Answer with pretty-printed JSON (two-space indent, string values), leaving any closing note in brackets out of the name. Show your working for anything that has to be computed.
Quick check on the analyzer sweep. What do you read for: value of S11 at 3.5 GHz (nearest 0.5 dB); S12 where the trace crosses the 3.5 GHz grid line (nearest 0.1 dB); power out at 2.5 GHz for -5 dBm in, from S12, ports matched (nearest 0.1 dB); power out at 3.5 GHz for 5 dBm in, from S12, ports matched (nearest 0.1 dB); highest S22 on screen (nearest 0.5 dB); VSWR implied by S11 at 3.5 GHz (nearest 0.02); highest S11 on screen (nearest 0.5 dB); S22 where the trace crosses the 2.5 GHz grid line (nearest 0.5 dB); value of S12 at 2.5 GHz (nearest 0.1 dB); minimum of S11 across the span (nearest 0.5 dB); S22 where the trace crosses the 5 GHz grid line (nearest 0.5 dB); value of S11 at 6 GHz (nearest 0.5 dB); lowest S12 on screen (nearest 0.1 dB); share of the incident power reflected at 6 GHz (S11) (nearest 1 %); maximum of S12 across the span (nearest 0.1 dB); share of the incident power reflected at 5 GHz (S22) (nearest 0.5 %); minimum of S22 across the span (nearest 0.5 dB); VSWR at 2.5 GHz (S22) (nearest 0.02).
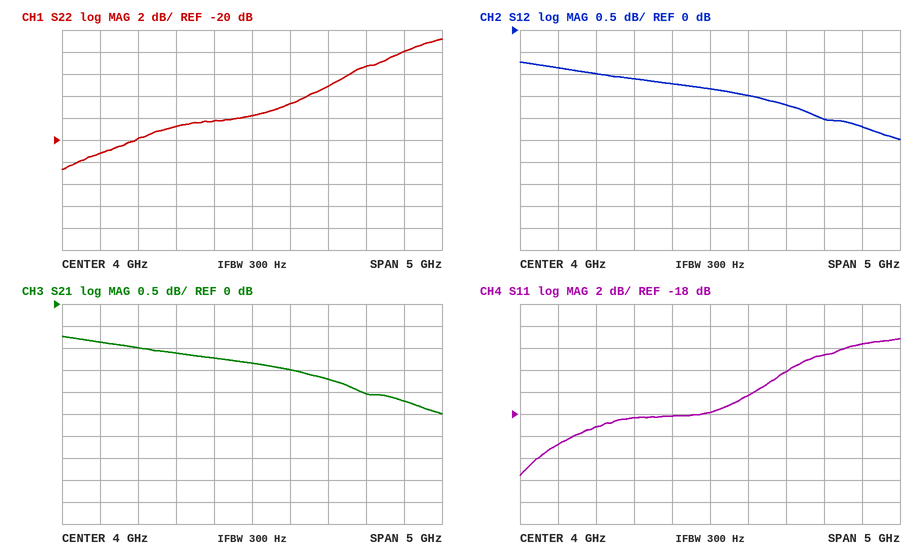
{
  "value of S11 at 3.5 GHz": "-18.0 dB",
  "S12 where the trace crosses the 3.5 GHz grid line": "-1.2 dB",
  "power out at 2.5 GHz for -5 dBm in, from S12, ports matched": "-5 dBm + (-1.0 dB) = -6.0 dBm",
  "power out at 3.5 GHz for 5 dBm in, from S12, ports matched": "5 dBm + (-1.2 dB) = 3.8 dBm",
  "highest S22 on screen": "-11.0 dB",
  "VSWR implied by S11 at 3.5 GHz": "|Γ| = 10^(-18/20) = 0.1259; VSWR = (1 + 0.1259)/(1 − 0.1259) ≈ 1.29, so 1.28 to the nearest 0.02",
  "highest S11 on screen": "-11.0 dB",
  "S22 where the trace crosses the 2.5 GHz grid line": "-20.0 dB",
  "value of S12 at 2.5 GHz": "-1.0 dB",
  "minimum of S11 across the span": "-23.5 dB",
  "S22 where the trace crosses the 5 GHz grid line": "-15.0 dB",
  "value of S11 at 6 GHz": "-11.5 dB",
  "lowest S12 on screen": "-2.5 dB",
  "share of the incident power reflected at 6 GHz (S11)": "10^(-11.5/10) ≈ 7 %",
  "maximum of S12 across the span": "-0.7 dB",
  "share of the incident power reflected at 5 GHz (S22)": "10^(-15/10) ≈ 3.16 %, so 3.0 % to the nearest 0.5 %",
  "minimum of S22 across the span": "-22.5 dB",
  "VSWR at 2.5 GHz (S22)": "|Γ| = 10^(-20/20) = 0.1000; VSWR = (1 + 0.1000)/(1 − 0.1000) ≈ 1.22"
}
